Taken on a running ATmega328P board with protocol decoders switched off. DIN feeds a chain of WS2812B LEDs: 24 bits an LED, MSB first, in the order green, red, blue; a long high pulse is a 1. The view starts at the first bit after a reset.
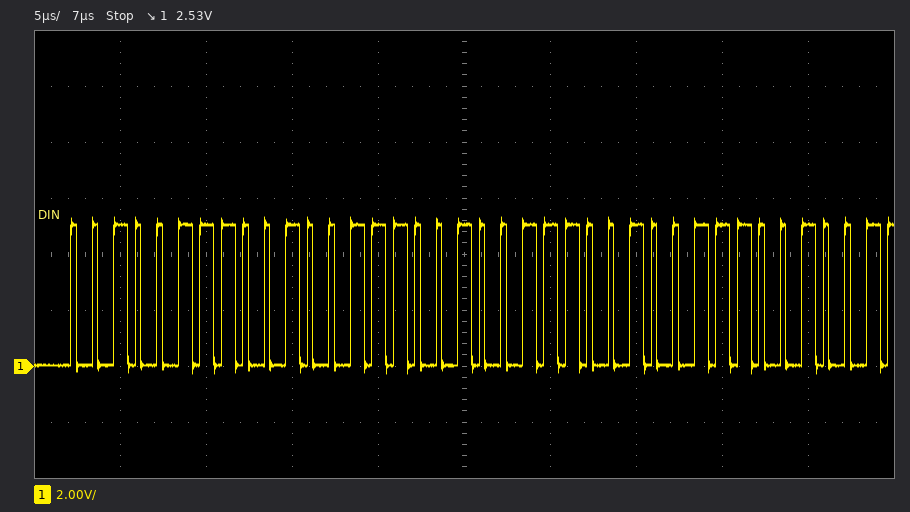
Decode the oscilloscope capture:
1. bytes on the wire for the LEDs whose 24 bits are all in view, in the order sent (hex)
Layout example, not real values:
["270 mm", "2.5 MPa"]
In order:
["27 27 27"]
